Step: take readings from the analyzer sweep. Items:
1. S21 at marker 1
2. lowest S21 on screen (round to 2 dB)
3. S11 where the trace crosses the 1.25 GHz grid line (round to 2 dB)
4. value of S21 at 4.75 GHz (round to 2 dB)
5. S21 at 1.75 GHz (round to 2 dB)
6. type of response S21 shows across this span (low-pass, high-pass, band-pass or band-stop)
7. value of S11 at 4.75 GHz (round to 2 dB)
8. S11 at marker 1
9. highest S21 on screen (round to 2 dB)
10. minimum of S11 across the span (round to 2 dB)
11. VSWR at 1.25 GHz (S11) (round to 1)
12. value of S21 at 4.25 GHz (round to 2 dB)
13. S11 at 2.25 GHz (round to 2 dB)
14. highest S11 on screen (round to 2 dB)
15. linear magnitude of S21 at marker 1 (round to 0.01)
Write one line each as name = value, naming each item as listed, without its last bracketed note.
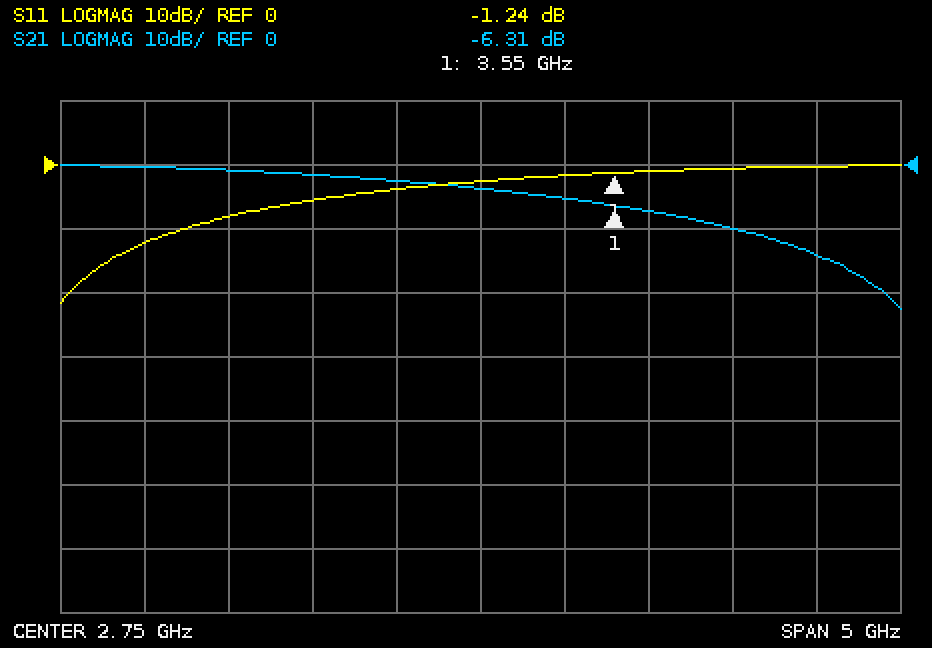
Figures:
S21 at marker 1 = -6.31 dB
lowest S21 on screen = -22 dB
S11 where the trace crosses the 1.25 GHz grid line = -8 dB
value of S21 at 4.75 GHz = -14 dB
S21 at 1.75 GHz = -2 dB
type of response S21 shows across this span = low-pass
value of S11 at 4.75 GHz = 0 dB
S11 at marker 1 = -1.24 dB
highest S21 on screen = 0 dB
minimum of S11 across the span = -22 dB
VSWR at 1.25 GHz (S11) = 2
value of S21 at 4.25 GHz = -10 dB
S11 at 2.25 GHz = -4 dB
highest S11 on screen = 0 dB
linear magnitude of S21 at marker 1 = 0.48
